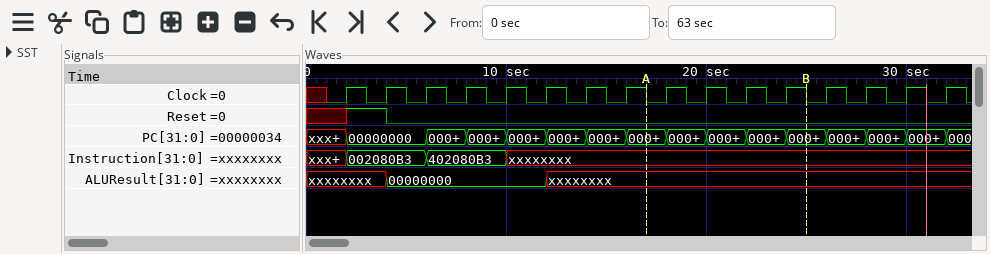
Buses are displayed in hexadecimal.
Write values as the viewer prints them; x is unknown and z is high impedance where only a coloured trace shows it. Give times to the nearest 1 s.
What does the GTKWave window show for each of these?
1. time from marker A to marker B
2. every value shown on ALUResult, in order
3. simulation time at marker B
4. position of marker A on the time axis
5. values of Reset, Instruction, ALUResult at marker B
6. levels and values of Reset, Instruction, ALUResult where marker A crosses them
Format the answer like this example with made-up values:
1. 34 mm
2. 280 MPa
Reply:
1. 8 s
2. xxxxxxxx, 00000000, xxxxxxxx
3. 25 s
4. 17 s
5. Reset=0, Instruction=xxxxxxxx, ALUResult=xxxxxxxx
6. Reset=0, Instruction=xxxxxxxx, ALUResult=xxxxxxxx
